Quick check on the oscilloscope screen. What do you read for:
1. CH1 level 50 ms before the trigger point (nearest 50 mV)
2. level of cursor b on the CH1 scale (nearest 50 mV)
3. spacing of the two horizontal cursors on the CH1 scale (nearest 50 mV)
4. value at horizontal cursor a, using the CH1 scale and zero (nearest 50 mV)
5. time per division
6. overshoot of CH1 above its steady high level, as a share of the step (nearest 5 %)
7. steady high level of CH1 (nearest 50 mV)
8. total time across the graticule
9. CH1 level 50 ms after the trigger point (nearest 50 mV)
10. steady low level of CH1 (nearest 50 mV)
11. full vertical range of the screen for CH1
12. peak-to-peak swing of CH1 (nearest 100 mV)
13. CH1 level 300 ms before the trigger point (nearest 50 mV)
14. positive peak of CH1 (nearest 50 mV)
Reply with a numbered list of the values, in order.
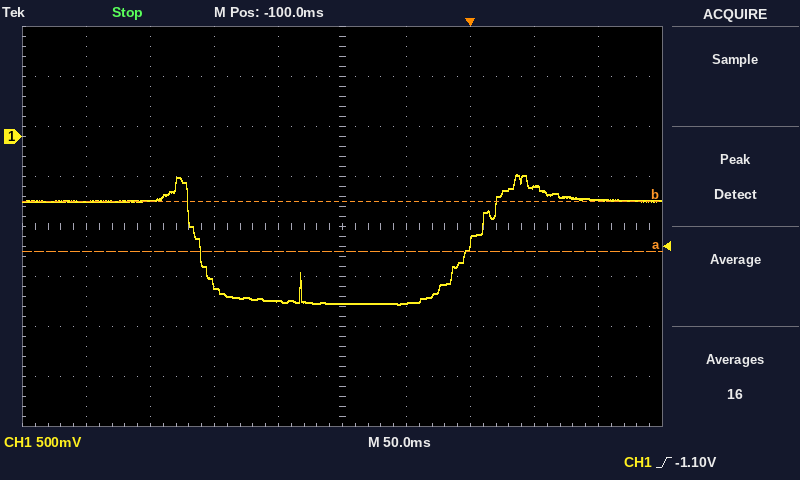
1. -1.65 V
2. -650 mV
3. 500 mV
4. -1.15 V
5. 50 ms
6. 25 %
7. -650 mV
8. 500 ms
9. -500 mV
10. -1.65 V
11. 4 V
12. 1.30 V
13. -650 mV
14. -400 mV
